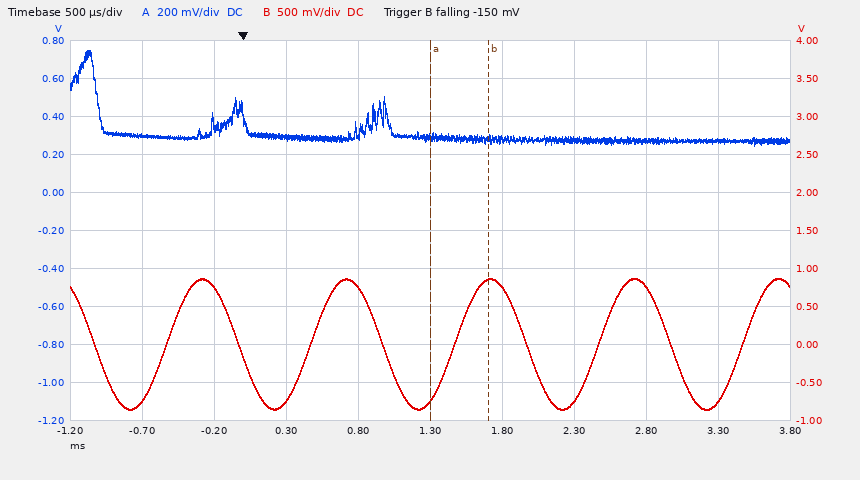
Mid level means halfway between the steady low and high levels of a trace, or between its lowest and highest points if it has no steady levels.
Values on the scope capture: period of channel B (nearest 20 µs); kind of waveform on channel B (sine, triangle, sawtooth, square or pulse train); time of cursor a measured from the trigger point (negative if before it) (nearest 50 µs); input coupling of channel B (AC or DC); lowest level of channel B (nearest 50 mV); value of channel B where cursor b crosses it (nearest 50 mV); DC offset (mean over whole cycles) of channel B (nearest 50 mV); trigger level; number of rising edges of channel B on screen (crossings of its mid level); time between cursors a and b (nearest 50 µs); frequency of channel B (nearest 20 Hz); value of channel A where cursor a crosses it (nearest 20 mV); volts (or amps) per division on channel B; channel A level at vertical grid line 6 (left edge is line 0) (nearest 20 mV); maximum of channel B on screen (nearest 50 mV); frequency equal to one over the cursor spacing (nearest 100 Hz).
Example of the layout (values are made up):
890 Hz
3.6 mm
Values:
1.00 ms
sine
+1.30 ms
DC
-850 mV
850 mV
0 mV
-150 mV
5
400 µs
1.00 kHz
300 mV
500 mV
280 mV
850 mV
2.5 kHz
